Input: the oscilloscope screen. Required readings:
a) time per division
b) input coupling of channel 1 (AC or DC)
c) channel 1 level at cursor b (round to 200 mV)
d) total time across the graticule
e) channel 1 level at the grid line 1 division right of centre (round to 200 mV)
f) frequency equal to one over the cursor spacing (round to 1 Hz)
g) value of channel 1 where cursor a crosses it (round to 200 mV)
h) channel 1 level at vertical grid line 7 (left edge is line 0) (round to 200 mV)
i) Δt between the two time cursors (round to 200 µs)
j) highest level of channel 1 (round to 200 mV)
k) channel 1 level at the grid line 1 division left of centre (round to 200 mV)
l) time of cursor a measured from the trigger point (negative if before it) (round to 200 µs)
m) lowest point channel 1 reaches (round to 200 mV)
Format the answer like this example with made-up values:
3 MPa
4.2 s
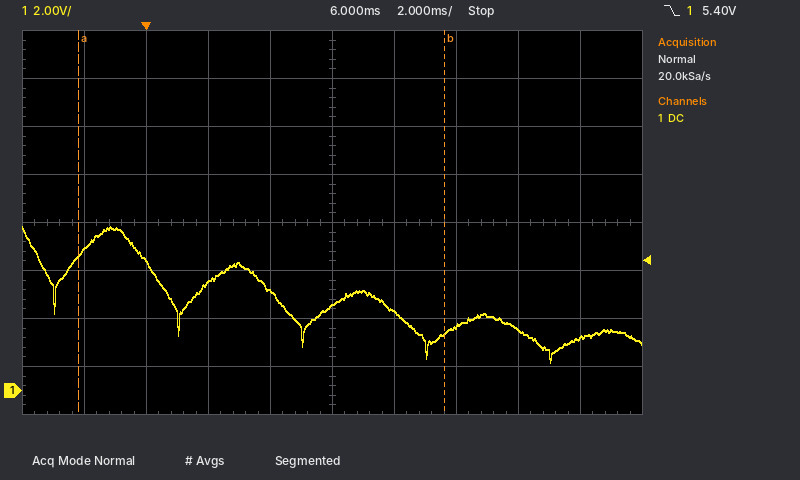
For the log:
2 ms
DC
2.4 V
20 ms
3.2 V
85 Hz
5.6 V
2.6 V
11.8 ms
6.8 V
4.2 V
-2.2 ms
1.2 V
